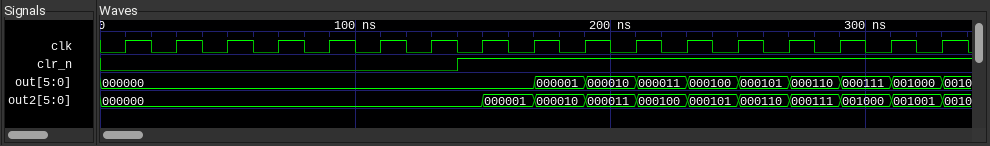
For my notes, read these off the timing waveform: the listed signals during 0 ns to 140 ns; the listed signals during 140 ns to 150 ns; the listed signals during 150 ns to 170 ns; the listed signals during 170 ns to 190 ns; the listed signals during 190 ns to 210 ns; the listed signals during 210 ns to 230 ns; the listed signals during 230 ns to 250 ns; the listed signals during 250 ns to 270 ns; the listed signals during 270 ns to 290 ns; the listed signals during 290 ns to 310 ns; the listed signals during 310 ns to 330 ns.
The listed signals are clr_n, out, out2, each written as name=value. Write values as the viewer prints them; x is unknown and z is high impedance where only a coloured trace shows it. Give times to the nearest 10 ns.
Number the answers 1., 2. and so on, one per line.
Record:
1. clr_n=0, out=000000, out2=000000
2. clr_n=1, out=000000, out2=000000
3. clr_n=1, out=000000, out2=000001
4. clr_n=1, out=000001, out2=000010
5. clr_n=1, out=000010, out2=000011
6. clr_n=1, out=000011, out2=000100
7. clr_n=1, out=000100, out2=000101
8. clr_n=1, out=000101, out2=000110
9. clr_n=1, out=000110, out2=000111
10. clr_n=1, out=000111, out2=001000
11. clr_n=1, out=001000, out2=001001
